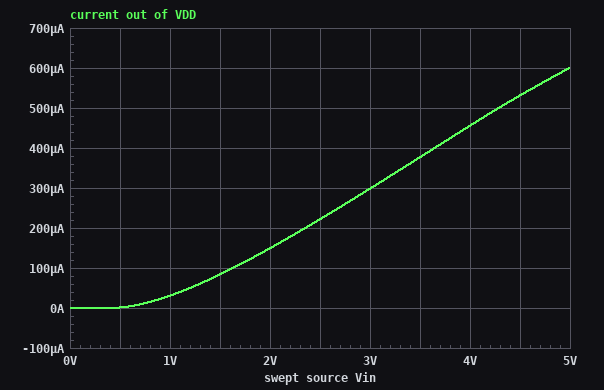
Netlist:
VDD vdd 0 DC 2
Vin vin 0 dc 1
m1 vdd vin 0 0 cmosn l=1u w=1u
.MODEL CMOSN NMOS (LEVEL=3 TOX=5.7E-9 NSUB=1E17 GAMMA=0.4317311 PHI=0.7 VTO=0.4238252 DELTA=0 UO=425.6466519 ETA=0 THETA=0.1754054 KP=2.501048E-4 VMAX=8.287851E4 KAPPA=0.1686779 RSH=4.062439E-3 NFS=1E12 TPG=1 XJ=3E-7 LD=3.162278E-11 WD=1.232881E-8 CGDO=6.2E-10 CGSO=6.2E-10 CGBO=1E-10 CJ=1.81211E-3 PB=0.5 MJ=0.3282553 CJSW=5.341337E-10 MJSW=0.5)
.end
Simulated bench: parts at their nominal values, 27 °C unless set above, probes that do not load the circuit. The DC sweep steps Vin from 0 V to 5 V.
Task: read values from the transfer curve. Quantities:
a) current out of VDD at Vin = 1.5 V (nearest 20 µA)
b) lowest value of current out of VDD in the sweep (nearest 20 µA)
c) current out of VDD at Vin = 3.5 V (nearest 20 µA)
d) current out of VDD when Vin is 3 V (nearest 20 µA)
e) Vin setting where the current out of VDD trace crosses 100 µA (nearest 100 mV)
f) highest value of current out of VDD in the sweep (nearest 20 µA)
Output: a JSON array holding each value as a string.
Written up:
["80 µA", "0 A", "380 µA", "300 µA", "1.6 V", "600 µA"]
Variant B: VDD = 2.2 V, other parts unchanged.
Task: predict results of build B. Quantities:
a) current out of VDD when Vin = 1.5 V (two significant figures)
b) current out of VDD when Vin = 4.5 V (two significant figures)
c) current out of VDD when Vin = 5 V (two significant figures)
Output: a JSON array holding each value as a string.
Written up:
["84 µA", "540 µA", "620 µA"]
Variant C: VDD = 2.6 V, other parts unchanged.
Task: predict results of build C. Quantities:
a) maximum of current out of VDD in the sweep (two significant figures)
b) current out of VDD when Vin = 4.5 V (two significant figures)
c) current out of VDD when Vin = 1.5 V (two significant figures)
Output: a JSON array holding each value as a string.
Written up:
["630 µA", "550 µA", "85 µA"]
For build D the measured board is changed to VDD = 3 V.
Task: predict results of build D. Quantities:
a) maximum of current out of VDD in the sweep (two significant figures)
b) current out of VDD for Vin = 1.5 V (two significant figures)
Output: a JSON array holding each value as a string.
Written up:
["640 µA", "86 µA"]
